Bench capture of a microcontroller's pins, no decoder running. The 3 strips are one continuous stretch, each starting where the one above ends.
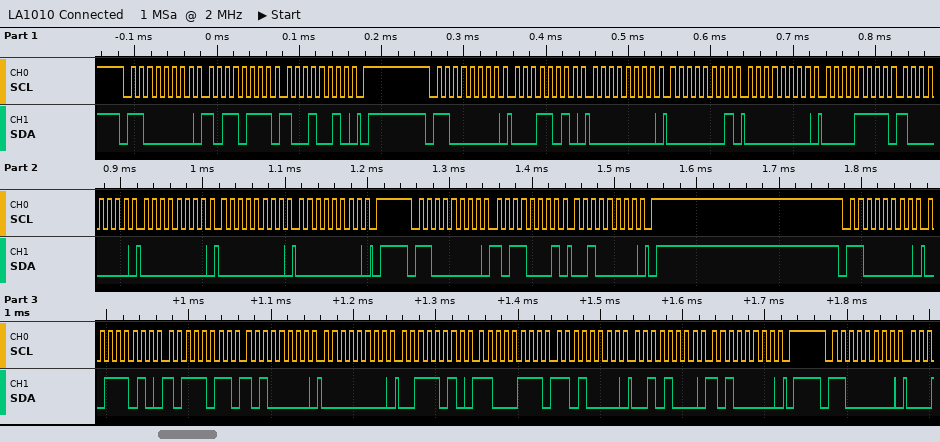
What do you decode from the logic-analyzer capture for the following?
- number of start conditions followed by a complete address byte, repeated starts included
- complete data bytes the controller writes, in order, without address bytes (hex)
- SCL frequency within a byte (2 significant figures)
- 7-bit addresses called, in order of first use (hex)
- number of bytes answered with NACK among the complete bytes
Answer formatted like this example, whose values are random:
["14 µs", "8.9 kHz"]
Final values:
["5", "B7 92 1A 00 01 00 0F 80 00 00 00 B1 20 3A BB A0 00 3A C7 D0 28 A0", "100 kHz", "0x60", "0"]
